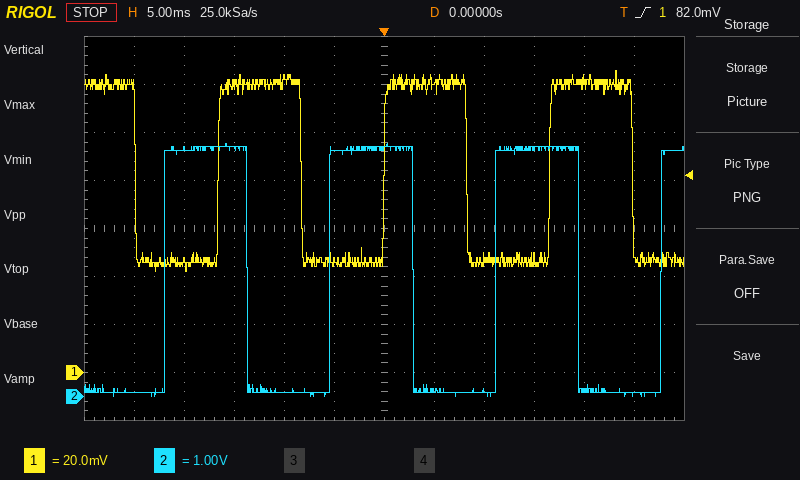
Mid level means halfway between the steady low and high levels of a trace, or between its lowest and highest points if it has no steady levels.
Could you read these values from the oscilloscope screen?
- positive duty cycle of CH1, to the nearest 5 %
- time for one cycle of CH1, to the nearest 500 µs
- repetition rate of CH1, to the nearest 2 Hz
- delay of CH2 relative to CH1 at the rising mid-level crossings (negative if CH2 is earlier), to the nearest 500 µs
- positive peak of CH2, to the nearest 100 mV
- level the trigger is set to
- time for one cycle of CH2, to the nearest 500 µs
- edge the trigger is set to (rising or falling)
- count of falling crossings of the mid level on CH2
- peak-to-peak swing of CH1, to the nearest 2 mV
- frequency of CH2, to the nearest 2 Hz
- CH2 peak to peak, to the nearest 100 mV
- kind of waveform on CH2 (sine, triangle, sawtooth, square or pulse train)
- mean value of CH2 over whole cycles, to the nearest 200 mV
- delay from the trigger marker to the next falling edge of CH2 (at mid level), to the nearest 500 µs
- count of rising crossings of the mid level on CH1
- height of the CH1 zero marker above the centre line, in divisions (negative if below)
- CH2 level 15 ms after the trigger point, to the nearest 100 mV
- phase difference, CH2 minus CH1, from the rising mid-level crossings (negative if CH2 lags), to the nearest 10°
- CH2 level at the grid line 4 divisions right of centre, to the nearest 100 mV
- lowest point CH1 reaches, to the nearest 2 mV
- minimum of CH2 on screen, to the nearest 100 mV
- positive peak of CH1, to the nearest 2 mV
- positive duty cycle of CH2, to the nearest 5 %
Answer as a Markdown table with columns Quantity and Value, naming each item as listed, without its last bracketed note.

| Quantity | Value |
|---|---|
| positive duty cycle of CH1, to the nearest 5 % | 50 % |
| time for one cycle of CH1, to the nearest 500 µs | 16.5 ms |
| repetition rate of CH1, to the nearest 2 Hz | 60 Hz |
| delay of CH2 relative to CH1 at the rising mid-level crossings (negative if CH2 is earlier), to the nearest 500 µs | -5.5 ms |
| positive peak of CH2, to the nearest 100 mV | 5.3 V |
| level the trigger is set to | 82.0 mV |
| time for one cycle of CH2, to the nearest 500 µs | 16.5 ms |
| edge the trigger is set to | rising |
| count of falling crossings of the mid level on CH2 | 3 |
| peak-to-peak swing of CH1, to the nearest 2 mV | 84 mV |
| frequency of CH2, to the nearest 2 Hz | 60 Hz |
| CH2 peak to peak, to the nearest 100 mV | 5.3 V |
| kind of waveform on CH2 | square |
| mean value of CH2 over whole cycles, to the nearest 200 mV | 2.6 V |
| delay from the trigger marker to the next falling edge of CH2 (at mid level), to the nearest 500 µs | 3.0 ms |
| count of rising crossings of the mid level on CH1 | 3 |
| height of the CH1 zero marker above the centre line, in divisions | -3.0 div |
| CH2 level 15 ms after the trigger point, to the nearest 100 mV | 5.2 V |
| phase difference, CH2 minus CH1, from the rising mid-level crossings (negative if CH2 lags), to the nearest 10° | +120° |
| CH2 level at the grid line 4 divisions right of centre, to the nearest 100 mV | 100 mV |
| lowest point CH1 reaches, to the nearest 2 mV | 42 mV |
| minimum of CH2 on screen, to the nearest 100 mV | 0.0 V |
| positive peak of CH1, to the nearest 2 mV | 126 mV |
| positive duty cycle of CH2, to the nearest 5 % | 50 % |
